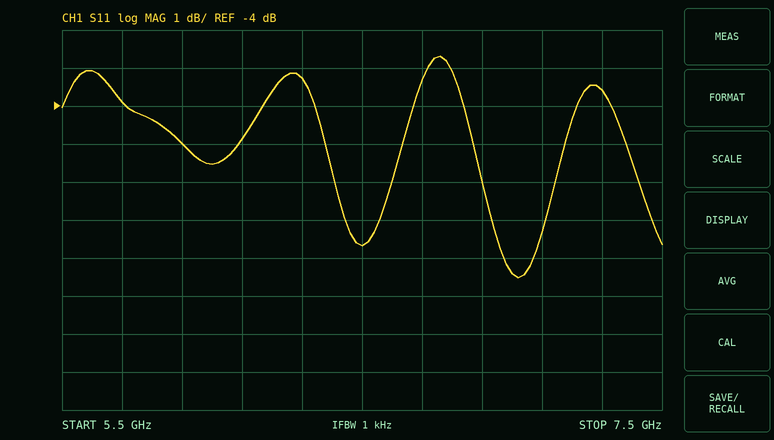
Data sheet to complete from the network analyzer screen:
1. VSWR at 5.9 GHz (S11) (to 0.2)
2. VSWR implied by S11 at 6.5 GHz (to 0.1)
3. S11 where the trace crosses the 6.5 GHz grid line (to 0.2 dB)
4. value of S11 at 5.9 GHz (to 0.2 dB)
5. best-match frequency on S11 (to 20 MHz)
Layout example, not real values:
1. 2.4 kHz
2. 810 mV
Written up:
1. 3.6
2. 2.4
3. -7.6 dB
4. -5.0 dB
5. 7.02 GHz
